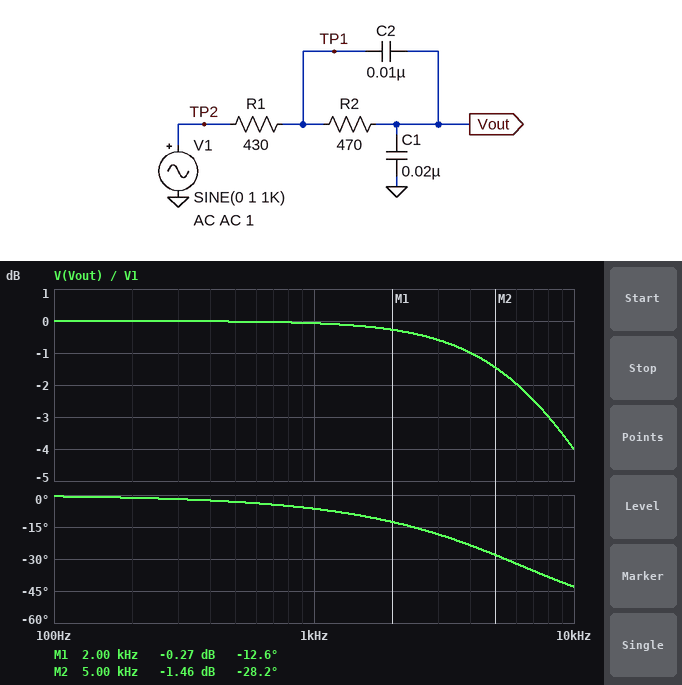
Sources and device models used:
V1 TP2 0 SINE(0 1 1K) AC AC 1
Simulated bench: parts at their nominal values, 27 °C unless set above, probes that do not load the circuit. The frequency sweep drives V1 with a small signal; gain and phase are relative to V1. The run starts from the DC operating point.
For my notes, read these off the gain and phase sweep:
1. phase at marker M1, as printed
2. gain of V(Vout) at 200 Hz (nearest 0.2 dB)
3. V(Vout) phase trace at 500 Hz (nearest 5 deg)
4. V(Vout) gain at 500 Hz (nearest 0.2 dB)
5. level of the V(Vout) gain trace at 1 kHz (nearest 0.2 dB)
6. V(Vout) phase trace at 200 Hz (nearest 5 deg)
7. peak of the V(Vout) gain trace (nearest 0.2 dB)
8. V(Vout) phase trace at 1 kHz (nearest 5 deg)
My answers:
-12.6 deg
0 dB
-5 deg
0 dB
0 dB
0 deg
0 dB
-5 deg
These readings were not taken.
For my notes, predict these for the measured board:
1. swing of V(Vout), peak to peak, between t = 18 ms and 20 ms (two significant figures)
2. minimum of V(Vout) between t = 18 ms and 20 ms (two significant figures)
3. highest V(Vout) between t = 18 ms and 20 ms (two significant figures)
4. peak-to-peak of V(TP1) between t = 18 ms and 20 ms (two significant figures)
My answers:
2.0 V
-990 mV
990 mV
2.0 V
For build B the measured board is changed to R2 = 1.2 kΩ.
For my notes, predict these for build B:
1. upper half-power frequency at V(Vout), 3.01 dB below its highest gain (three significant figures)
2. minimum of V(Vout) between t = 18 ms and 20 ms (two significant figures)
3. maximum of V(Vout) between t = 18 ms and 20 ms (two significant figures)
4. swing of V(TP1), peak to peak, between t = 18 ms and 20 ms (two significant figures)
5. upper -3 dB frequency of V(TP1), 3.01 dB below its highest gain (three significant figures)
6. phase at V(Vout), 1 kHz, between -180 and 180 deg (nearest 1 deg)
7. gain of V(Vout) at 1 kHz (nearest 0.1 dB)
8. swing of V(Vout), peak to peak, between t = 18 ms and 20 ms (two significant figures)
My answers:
4.11 kHz
-970 mV
970 mV
2.0 V
44.2 kHz
-11 deg
-0.3 dB
1.9 V
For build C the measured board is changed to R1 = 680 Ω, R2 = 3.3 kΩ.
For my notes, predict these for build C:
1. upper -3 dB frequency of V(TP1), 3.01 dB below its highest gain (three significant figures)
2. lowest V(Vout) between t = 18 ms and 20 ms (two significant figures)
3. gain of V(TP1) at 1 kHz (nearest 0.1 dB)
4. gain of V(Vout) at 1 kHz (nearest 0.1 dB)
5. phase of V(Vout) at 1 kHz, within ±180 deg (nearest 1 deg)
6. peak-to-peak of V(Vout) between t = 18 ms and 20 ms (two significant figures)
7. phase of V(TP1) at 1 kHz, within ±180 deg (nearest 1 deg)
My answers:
31.4 kHz
-840 mV
-0.2 dB
-1.5 dB
-24 deg
1.7 V
-4 deg
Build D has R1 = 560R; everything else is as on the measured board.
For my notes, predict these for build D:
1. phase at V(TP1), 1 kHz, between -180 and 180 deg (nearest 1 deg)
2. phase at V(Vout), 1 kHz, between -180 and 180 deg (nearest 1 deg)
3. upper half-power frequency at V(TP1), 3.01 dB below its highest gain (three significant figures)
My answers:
-4 deg
-7 deg
12.8 kHz
